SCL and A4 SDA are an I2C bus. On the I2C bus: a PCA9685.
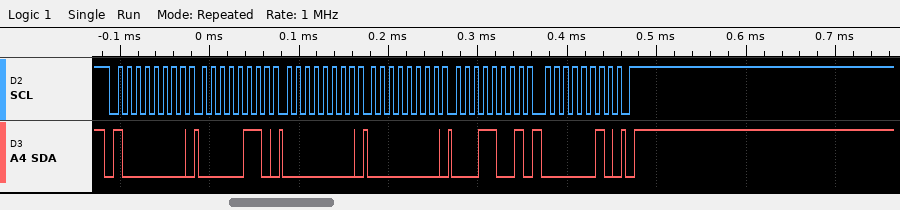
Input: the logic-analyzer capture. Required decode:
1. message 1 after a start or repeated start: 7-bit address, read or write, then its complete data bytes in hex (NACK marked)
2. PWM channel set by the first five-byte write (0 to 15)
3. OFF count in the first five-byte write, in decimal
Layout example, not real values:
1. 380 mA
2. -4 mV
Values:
1. 0x40 write: 06 00 00 19 02
2. 0
3. 537
